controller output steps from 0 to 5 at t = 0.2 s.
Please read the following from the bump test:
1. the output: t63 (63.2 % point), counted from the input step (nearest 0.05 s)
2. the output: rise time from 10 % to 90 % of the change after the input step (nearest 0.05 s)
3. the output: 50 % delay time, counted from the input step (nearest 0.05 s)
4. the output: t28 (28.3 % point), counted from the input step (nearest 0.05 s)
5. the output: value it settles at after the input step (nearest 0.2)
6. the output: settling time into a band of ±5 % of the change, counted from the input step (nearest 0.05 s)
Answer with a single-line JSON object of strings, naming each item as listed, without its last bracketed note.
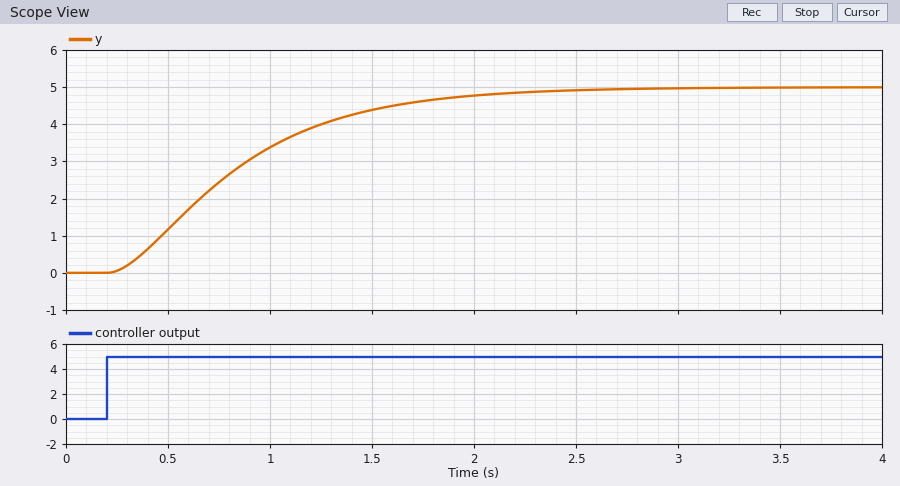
{"the output: t63 (63.2 % point), counted from the input step": "0.75 s", "the output: rise time from 10 % to 90 % of the change after the input step": "1.25 s", "the output: 50 % delay time, counted from the input step": "0.55 s", "the output: t28 (28.3 % point), counted from the input step": "0.35 s", "the output: value it settles at after the input step": "5.0", "the output: settling time into a band of ±5 % of the change, counted from the input step": "1.75 s"}
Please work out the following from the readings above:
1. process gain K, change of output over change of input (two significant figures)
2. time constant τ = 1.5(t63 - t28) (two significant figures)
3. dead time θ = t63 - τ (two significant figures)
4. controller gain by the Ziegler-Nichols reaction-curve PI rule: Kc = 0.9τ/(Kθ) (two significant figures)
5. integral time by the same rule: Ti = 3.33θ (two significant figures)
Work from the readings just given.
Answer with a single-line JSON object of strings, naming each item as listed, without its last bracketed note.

{"process gain K, change of output over change of input": "1.0", "time constant τ = 1.5(t63 - t28)": "0.60 s", "dead time θ = t63 - τ": "0.15 s", "controller gain by the Ziegler-Nichols reaction-curve PI rule: Kc = 0.9τ/(Kθ)": "3.6", "integral time by the same rule: Ti = 3.33θ": "0.50 s"}
